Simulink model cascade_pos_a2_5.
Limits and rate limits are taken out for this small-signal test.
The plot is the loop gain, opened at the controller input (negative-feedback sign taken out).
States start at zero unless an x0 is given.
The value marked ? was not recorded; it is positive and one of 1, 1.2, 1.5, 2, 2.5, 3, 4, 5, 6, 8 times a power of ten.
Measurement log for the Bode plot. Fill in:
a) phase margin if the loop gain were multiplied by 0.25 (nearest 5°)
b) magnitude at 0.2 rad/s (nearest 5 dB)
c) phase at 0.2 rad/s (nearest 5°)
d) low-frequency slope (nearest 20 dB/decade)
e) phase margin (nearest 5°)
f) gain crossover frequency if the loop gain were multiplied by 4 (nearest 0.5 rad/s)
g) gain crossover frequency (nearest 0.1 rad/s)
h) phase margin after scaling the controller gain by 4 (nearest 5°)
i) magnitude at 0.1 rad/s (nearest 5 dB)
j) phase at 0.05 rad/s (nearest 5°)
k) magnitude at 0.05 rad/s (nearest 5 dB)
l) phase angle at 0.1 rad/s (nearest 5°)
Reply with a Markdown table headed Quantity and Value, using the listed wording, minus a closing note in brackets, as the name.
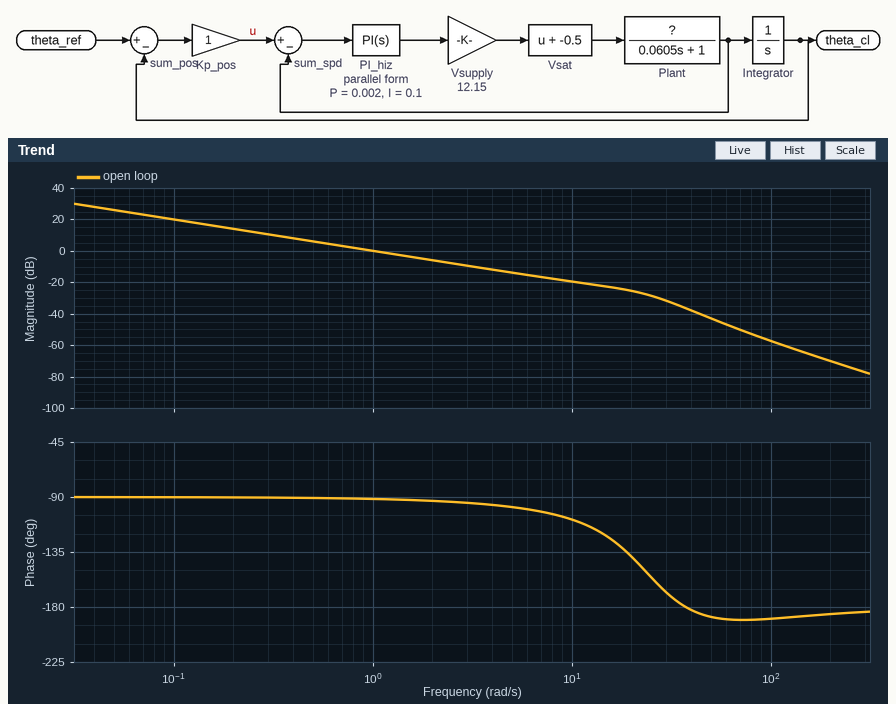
| Quantity | Value |
|---|---|
| phase margin if the loop gain were multiplied by 0.25 | 90° |
| magnitude at 0.2 rad/s | 15 dB |
| phase at 0.2 rad/s | -90° |
| low-frequency slope | -20 dB/decade |
| phase margin | 90° |
| gain crossover frequency if the loop gain were multiplied by 4 | 4.0 rad/s |
| gain crossover frequency | 1.0 rad/s |
| phase margin after scaling the controller gain by 4 | 85° |
| magnitude at 0.1 rad/s | 20 dB |
| phase at 0.05 rad/s | -90° |
| magnitude at 0.05 rad/s | 25 dB |
| phase angle at 0.1 rad/s | -90° |
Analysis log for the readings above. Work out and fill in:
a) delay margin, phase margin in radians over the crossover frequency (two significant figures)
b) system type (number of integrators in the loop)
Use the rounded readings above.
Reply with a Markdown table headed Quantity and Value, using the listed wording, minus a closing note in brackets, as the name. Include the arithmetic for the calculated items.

| Quantity | Value |
|---|---|
| delay margin, phase margin in radians over the crossover frequency | 90 × π / 180 / 1 = 1.6 s |
| system type | 1 |
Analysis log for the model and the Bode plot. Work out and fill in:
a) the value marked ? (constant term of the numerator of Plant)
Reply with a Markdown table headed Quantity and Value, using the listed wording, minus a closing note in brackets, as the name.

| Quantity | Value |
|---|---|
| the value marked ? | 30 |
